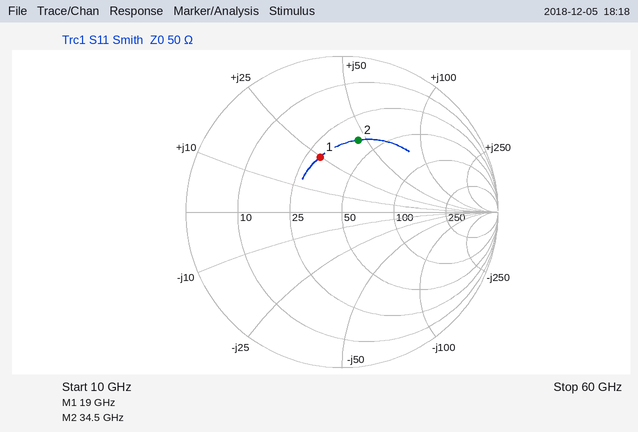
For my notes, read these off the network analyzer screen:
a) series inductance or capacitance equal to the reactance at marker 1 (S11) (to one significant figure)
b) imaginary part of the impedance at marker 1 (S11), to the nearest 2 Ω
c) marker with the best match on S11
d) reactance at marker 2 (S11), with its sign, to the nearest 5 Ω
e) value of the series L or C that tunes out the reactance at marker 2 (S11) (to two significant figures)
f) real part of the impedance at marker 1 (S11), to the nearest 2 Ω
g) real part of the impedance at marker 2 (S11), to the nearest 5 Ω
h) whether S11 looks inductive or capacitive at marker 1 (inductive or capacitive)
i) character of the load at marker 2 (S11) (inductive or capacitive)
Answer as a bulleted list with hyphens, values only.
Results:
- 200 pH
- +24 Ω
- marker 1
- +45 Ω
- 100 fF
- 30 Ω
- 40 Ω
- inductive
- inductive
